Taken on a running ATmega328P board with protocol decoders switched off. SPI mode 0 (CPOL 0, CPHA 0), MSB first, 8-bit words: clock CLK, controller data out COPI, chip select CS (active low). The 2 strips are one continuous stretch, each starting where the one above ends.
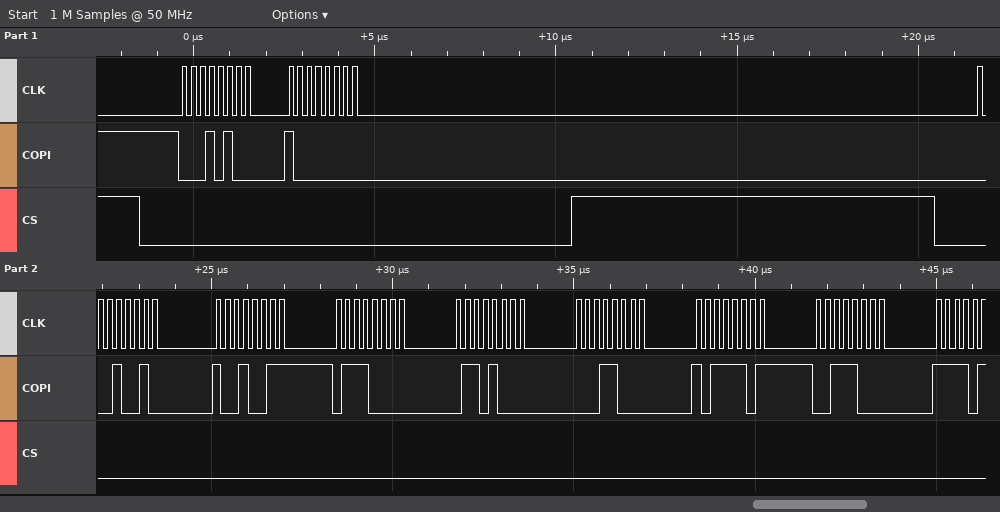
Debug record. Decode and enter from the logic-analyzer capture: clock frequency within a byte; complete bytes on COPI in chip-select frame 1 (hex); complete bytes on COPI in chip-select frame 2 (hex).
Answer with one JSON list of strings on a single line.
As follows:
["4 MHz", "14 80", "12 93 70 68 18 BD 38"]
